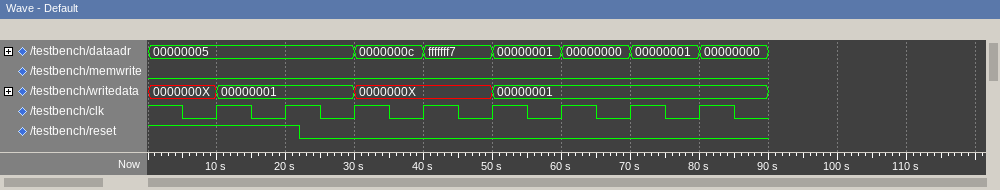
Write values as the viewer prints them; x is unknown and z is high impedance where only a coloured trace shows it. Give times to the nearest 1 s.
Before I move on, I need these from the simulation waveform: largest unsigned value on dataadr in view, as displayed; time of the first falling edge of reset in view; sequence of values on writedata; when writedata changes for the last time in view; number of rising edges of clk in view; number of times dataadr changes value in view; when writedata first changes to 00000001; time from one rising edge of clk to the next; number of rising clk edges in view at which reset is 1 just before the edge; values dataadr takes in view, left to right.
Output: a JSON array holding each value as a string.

["fffffff7", "22 s", "0000000X, 00000001, 0000000X, 00000001", "50 s", "8", "6", "10 s", "10 s", "2", "00000005, 0000000c, fffffff7, 00000001, 00000000, 00000001, 00000000"]
